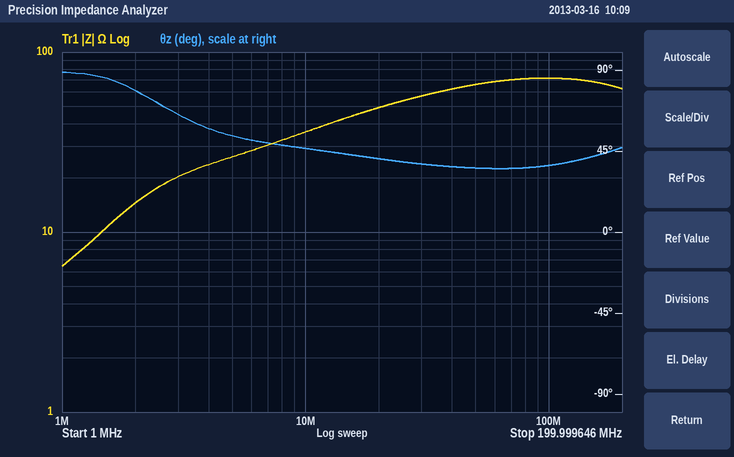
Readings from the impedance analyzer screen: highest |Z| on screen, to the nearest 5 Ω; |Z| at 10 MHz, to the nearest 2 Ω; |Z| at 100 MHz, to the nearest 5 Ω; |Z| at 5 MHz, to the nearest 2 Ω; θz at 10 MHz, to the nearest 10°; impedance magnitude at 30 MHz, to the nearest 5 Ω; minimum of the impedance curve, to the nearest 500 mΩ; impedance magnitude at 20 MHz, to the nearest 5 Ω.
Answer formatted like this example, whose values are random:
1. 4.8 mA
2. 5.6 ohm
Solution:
1. 70 Ω
2. 36 Ω
3. 70 Ω
4. 26 Ω
5. 50°
6. 55 Ω
7. 6.5 Ω
8. 50 Ω
